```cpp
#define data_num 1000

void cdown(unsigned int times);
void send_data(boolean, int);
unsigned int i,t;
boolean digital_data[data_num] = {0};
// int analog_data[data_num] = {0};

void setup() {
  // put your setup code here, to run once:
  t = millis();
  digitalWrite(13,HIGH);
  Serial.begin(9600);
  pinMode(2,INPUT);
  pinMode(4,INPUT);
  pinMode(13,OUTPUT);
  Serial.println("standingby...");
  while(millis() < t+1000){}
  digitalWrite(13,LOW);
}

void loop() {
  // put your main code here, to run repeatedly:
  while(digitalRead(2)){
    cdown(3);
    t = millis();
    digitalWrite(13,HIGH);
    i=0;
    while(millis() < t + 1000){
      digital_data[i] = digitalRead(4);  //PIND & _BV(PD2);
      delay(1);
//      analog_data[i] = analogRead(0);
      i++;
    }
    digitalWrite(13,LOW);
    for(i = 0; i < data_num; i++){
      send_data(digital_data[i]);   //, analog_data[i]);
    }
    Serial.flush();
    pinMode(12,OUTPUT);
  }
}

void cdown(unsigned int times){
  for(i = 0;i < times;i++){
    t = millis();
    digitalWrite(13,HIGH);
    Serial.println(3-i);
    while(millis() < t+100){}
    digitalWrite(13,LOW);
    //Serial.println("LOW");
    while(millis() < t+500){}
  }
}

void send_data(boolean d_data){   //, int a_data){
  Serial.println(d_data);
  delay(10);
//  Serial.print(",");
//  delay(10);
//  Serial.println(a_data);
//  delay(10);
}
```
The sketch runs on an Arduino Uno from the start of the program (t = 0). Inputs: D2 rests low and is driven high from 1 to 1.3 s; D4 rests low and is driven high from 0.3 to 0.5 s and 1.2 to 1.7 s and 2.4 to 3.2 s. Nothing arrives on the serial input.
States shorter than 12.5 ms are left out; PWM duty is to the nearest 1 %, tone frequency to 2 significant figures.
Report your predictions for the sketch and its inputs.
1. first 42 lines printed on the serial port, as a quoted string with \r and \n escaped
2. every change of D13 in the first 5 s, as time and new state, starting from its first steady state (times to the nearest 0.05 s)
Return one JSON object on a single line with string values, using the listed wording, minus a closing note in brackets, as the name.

{"first 42 lines printed on the serial port, as a quoted string with \\r and \\n escaped": "\"standingby...\\r\\n3\\r\\n2\\r\\n1\\r\\n1\\r\\n1\\r\\n1\\r\\n1\\r\\n1\\r\\n1\\r\\n1\\r\\n1\\r\\n1\\r\\n1\\r\\n1\\r\\n1\\r\\n1\\r\\n1\\r\\n1\\r\\n1\\r\\n1\\r\\n1\\r\\n1\\r\\n1\\r\\n1\\r\\n1\\r\\n1\\r\\n1\\r\\n1\\r\\n1\\r\\n1\\r\\n1\\r\\n1\\r\\n1\\r\\n1\\r\\n1\\r\\n1\\r\\n1\\r\\n1\\r\\n1\\r\\n1\\r\\n1\\r\\n\"", "every change of D13 in the first 5 s, as time and new state, starting from its first steady state": "0 s high; 1.1 s low; 1.5 s high; 1.6 s low; 2 s high; 2.1 s low; 2.5 s high; 3.5 s low"}
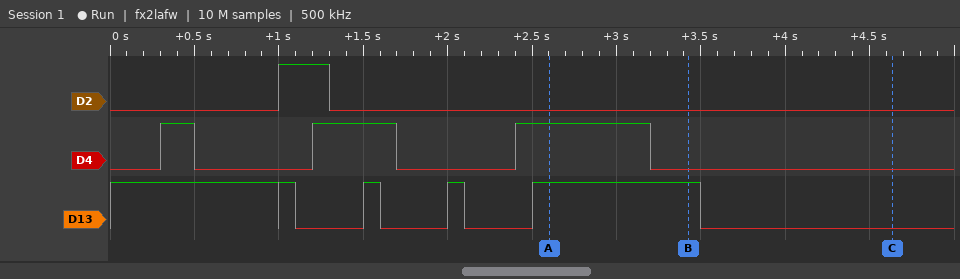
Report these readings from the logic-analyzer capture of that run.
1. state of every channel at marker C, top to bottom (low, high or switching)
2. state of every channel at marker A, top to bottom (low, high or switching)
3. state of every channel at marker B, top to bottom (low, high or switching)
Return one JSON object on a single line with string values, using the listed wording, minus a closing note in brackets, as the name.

{"state of every channel at marker C, top to bottom": "D2 low, D4 low, D13 low", "state of every channel at marker A, top to bottom": "D2 low, D4 high, D13 high", "state of every channel at marker B, top to bottom": "D2 low, D4 low, D13 high"}
